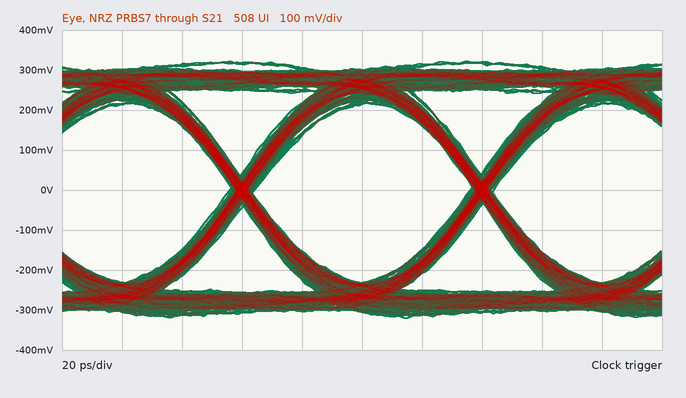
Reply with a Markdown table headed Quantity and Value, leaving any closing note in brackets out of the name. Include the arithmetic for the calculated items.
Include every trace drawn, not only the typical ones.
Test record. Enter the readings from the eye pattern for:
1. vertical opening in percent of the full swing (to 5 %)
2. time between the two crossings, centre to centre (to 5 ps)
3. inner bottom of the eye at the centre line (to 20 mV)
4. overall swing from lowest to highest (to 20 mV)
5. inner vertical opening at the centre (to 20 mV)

| Quantity | Value |
|---|---|
| vertical opening in percent of the full swing | 440 mV / 640 mV ≈ 68.8 %, so 70 % to the nearest 5 % |
| time between the two crossings, centre to centre | 80 ps |
| inner bottom of the eye at the centre line | -240 mV |
| overall swing from lowest to highest | 640 mV |
| inner vertical opening at the centre | 440 mV |
